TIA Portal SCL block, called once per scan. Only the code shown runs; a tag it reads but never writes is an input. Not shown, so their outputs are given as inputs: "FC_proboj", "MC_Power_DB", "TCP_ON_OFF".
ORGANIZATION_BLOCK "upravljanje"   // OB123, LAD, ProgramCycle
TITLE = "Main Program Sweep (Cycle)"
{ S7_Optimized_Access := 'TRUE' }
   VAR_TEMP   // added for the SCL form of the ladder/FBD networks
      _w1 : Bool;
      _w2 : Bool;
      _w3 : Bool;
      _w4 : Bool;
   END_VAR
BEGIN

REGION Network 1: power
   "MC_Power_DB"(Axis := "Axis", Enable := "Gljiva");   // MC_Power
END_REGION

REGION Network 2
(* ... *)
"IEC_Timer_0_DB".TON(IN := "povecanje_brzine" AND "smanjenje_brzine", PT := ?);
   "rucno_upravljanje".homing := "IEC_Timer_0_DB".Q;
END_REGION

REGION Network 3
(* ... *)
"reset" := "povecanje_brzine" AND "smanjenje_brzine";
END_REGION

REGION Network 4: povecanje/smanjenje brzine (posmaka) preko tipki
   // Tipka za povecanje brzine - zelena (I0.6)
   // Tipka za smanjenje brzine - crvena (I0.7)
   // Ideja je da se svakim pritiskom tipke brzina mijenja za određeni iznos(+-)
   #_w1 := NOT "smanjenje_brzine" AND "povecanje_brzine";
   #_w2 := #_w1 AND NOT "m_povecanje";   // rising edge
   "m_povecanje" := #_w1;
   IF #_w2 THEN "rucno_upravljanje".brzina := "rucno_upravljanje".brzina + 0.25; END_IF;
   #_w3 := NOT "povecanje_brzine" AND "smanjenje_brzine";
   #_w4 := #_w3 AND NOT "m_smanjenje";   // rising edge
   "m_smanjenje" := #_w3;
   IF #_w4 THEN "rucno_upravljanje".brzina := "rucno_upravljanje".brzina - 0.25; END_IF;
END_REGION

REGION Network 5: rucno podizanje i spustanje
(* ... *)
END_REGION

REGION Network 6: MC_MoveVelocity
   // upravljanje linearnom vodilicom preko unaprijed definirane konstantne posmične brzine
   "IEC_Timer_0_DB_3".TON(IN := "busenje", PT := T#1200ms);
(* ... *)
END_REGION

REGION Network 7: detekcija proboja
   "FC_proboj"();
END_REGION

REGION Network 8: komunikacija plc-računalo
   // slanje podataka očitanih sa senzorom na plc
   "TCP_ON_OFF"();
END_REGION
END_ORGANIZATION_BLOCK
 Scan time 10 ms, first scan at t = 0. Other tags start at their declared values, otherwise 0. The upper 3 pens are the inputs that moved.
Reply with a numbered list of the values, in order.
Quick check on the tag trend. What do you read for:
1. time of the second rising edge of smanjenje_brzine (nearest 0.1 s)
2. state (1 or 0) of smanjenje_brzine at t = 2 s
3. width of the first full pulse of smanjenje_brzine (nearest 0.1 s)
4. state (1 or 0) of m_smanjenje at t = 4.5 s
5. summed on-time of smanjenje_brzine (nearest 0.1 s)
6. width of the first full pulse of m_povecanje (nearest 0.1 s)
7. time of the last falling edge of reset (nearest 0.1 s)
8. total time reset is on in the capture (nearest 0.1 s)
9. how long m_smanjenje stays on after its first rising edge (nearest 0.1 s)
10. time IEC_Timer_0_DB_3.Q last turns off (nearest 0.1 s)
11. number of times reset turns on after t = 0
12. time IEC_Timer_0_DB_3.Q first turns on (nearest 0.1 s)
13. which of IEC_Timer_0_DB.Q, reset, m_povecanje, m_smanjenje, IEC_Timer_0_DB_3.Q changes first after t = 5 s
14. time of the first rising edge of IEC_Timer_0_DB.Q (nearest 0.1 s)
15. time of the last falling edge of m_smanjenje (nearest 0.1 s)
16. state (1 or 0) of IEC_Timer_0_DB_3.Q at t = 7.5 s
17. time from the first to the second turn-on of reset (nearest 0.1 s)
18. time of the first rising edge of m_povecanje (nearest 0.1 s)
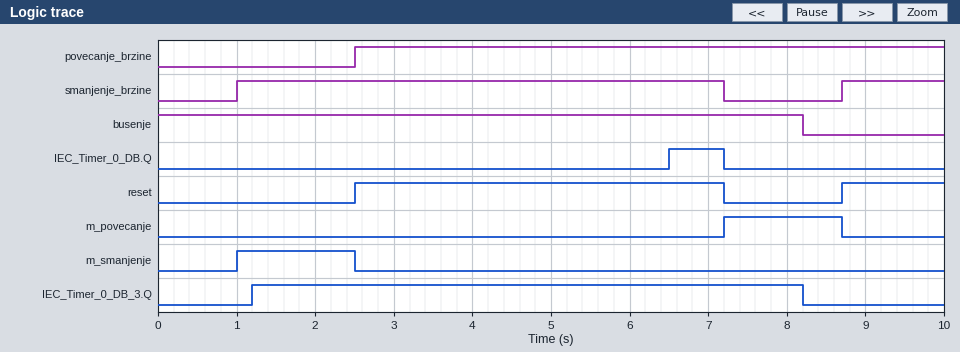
1. 8.7 s
2. 1
3. 6.2 s
4. 0
5. 7.5 s
6. 1.5 s
7. 7.2 s
8. 6.0 s
9. 1.5 s
10. 8.2 s
11. 2
12. 1.2 s
13. IEC_Timer_0_DB.Q
14. 6.5 s
15. 2.5 s
16. 1
17. 6.2 s
18. 7.2 s
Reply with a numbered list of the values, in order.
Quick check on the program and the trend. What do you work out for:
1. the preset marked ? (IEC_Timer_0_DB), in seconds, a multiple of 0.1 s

1. 4.0 s
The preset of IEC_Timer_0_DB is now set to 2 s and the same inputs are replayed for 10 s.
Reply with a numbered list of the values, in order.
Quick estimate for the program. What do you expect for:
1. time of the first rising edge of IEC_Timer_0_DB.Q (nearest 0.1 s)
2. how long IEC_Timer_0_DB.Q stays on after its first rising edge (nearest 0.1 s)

1. 4.5 s
2. 2.7 s
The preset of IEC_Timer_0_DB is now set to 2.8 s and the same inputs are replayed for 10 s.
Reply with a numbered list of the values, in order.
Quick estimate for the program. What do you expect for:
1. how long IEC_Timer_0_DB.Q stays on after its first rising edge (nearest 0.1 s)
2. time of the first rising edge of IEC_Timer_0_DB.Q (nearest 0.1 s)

1. 1.9 s
2. 5.3 s
